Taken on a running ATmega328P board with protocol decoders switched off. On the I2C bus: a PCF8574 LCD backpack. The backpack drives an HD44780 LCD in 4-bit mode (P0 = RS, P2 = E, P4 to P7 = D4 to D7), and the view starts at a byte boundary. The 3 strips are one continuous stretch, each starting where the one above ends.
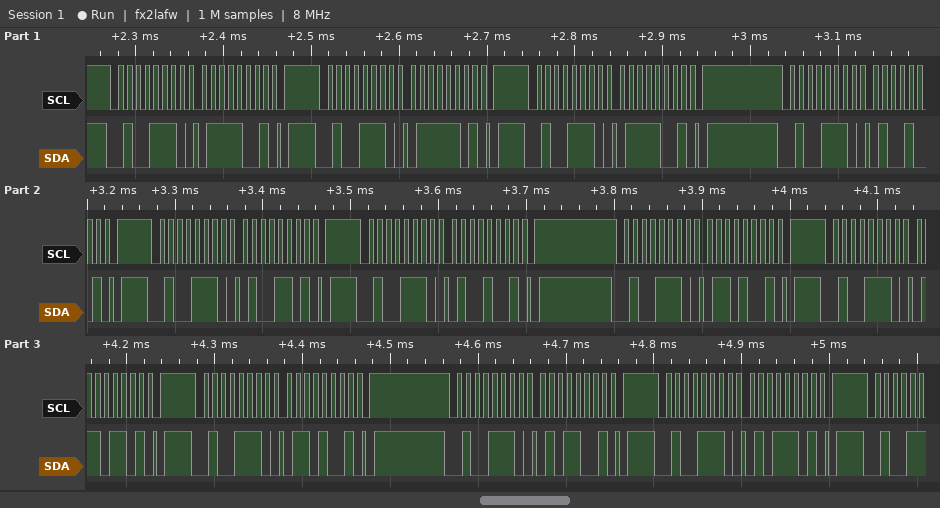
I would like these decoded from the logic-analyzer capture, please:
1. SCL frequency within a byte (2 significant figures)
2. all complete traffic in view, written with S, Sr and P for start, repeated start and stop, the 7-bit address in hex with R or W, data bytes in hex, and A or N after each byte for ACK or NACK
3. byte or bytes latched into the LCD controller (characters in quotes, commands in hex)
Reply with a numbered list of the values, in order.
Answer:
1. 100 kHz
2. S 27W A 79 A P S 27W A 7D A P S 27W A 79 A P S 27W A 49 A P S 27W A 4D A P S 27W A 49 A P S 27W A 69 A P S 27W A 6D A P S 27W A 69 A P S 27W A 59 A P S 27W A 5D A P
3. 't'
